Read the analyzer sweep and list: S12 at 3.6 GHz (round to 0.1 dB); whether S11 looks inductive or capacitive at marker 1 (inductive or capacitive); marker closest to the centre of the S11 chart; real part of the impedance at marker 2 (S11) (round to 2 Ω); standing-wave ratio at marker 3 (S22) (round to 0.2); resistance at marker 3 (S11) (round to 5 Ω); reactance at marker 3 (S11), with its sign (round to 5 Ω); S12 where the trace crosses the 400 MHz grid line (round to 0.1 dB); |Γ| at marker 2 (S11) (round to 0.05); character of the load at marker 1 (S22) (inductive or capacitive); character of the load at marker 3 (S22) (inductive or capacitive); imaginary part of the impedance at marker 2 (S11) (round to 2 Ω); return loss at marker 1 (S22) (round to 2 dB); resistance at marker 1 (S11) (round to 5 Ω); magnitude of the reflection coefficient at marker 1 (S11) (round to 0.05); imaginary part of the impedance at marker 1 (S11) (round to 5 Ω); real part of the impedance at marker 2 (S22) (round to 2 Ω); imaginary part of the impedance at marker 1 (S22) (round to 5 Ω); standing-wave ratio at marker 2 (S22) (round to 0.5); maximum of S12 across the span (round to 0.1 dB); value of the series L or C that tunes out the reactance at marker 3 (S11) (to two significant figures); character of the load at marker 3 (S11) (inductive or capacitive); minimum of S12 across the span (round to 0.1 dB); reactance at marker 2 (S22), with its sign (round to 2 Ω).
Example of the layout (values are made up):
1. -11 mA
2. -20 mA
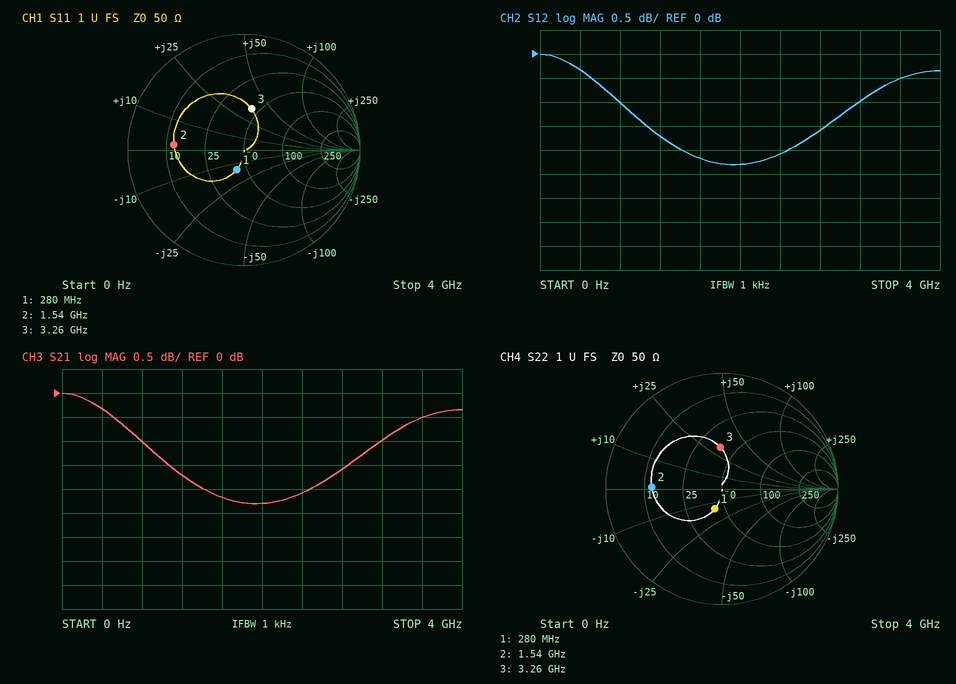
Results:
1. -0.5 dB
2. capacitive
3. marker 1
4. 12 Ω
5. 2.2
6. 45 Ω
7. +35 Ω
8. -0.3 dB
9. 0.60
10. capacitive
11. inductive
12. +2 Ω
13. 14 dB
14. 40 Ω
15. 0.20
16. -15 Ω
17. 12 Ω
18. -15 Ω
19. 4.0
20. 0.0 dB
21. 1.4 pF
22. inductive
23. -2.3 dB
24. 0 Ω
